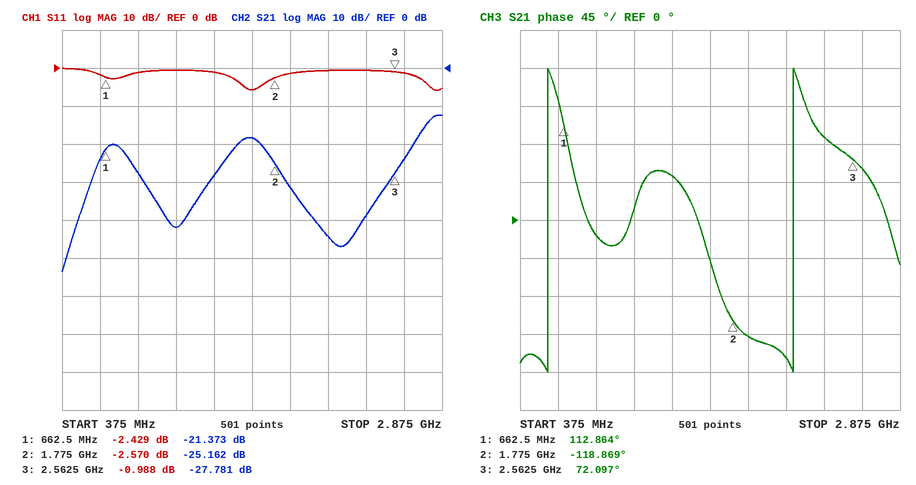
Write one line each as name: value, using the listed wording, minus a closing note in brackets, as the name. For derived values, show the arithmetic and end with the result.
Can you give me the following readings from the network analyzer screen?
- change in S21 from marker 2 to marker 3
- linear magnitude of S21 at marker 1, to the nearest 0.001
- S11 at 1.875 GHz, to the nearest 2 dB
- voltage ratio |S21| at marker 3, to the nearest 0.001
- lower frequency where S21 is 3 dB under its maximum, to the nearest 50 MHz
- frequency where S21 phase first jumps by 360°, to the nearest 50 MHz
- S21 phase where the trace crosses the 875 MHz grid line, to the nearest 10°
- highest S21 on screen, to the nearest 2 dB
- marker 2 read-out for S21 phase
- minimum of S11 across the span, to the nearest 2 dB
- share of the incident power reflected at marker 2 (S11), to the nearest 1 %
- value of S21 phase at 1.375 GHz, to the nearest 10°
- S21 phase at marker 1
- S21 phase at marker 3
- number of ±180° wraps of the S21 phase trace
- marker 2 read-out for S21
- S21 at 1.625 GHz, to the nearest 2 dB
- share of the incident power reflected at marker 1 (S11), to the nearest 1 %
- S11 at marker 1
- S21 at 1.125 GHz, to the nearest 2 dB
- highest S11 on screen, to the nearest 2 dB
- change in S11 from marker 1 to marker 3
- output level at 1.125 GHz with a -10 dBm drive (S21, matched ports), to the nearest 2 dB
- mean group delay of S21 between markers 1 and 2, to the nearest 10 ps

change in S21 from marker 2 to marker 3: -27.781 − (-25.162) = -2.619 dB
linear magnitude of S21 at marker 1, to the nearest 0.001: 10^(-21.373/20) ≈ 0.085
S11 at 1.875 GHz, to the nearest 2 dB: -2 dB
voltage ratio |S21| at marker 3, to the nearest 0.001: 10^(-27.781/20) ≈ 0.041
lower frequency where S21 is 3 dB under its maximum, to the nearest 50 MHz: 2.75 GHz
frequency where S21 phase first jumps by 360°, to the nearest 50 MHz: 550 MHz
S21 phase where the trace crosses the 875 MHz grid line, to the nearest 10°: -20°
highest S21 on screen, to the nearest 2 dB: -12 dB
marker 2 read-out for S21 phase: -118.869°
minimum of S11 across the span, to the nearest 2 dB: -6 dB
share of the incident power reflected at marker 2 (S11), to the nearest 1 %: 10^(-2.57/10) ≈ 55 %
value of S21 phase at 1.375 GHz, to the nearest 10°: 50°
S21 phase at marker 1: 112.864°
S21 phase at marker 3: 72.097°
number of ±180° wraps of the S21 phase trace: 2
marker 2 read-out for S21: -25.162 dB
S21 at 1.625 GHz, to the nearest 2 dB: -18 dB
share of the incident power reflected at marker 1 (S11), to the nearest 1 %: 10^(-2.429/10) ≈ 57 %
S11 at marker 1: -2.429 dB
S21 at 1.125 GHz, to the nearest 2 dB: -42 dB
highest S11 on screen, to the nearest 2 dB: 0 dB
change in S11 from marker 1 to marker 3: -0.988 − (-2.429) = 1.441 dB
output level at 1.125 GHz with a -10 dBm drive (S21, matched ports), to the nearest 2 dB: -10 dBm + (-42 dB) = -52 dBm
mean group delay of S21 between markers 1 and 2, to the nearest 10 ps: −(-118.869° − (112.864°))/(360° × 1.1125 GHz) ≈ 579 ps, so 580 ps to the nearest 10 ps
